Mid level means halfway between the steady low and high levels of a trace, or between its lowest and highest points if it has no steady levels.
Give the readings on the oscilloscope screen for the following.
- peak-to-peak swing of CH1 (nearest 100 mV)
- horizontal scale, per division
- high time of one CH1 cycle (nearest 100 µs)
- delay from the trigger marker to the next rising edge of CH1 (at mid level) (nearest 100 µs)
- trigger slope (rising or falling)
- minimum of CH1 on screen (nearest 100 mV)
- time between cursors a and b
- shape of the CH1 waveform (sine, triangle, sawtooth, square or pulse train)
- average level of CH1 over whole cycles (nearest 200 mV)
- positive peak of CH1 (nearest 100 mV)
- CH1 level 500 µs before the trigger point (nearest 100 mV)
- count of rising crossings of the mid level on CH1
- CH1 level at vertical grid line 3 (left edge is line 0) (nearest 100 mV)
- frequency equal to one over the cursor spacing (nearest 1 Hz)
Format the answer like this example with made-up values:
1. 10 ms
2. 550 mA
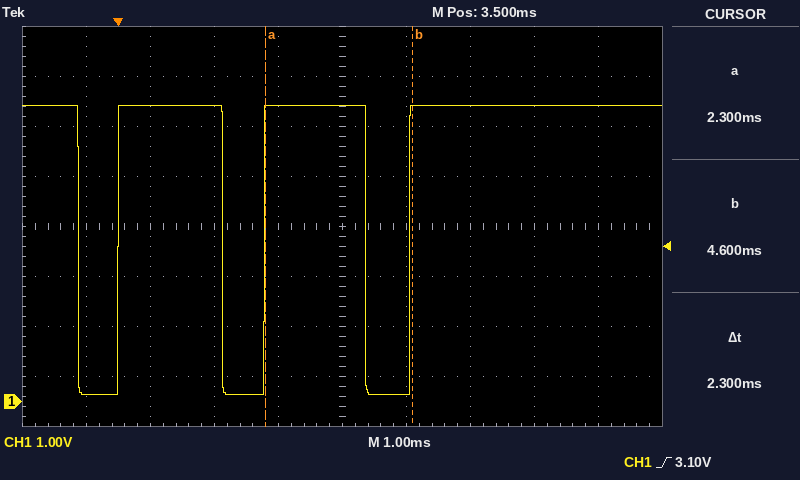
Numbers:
1. 5.8 V
2. 1 ms
3. 1.6 ms
4. 2.3 ms
5. rising
6. 100 mV
7. 2.3 ms
8. pulse train
9. 4.2 V
10. 5.9 V
11. 100 mV
12. 3
13. 5.9 V
14. 435 Hz
